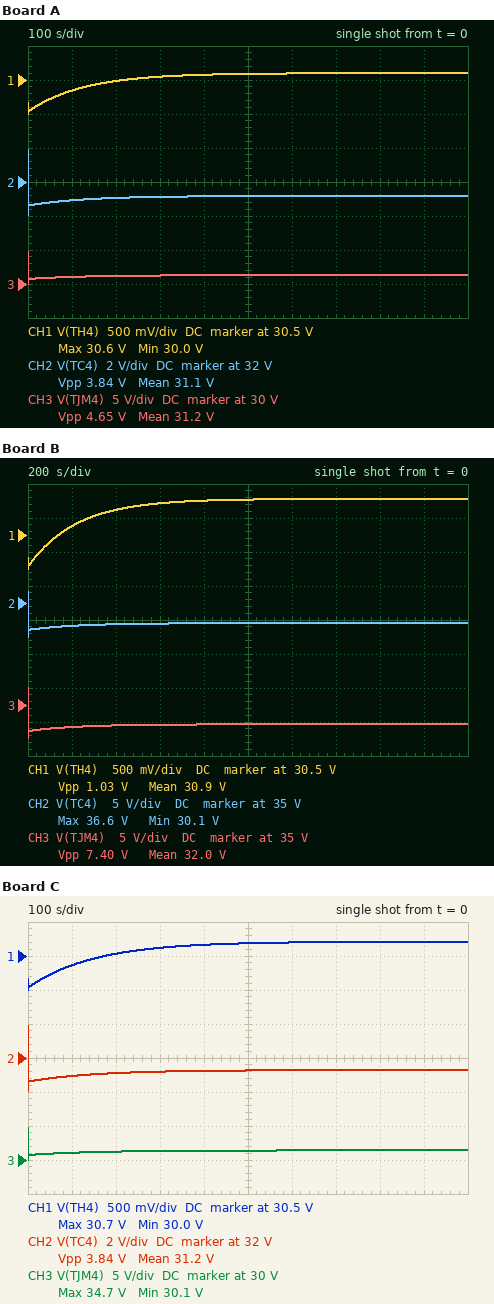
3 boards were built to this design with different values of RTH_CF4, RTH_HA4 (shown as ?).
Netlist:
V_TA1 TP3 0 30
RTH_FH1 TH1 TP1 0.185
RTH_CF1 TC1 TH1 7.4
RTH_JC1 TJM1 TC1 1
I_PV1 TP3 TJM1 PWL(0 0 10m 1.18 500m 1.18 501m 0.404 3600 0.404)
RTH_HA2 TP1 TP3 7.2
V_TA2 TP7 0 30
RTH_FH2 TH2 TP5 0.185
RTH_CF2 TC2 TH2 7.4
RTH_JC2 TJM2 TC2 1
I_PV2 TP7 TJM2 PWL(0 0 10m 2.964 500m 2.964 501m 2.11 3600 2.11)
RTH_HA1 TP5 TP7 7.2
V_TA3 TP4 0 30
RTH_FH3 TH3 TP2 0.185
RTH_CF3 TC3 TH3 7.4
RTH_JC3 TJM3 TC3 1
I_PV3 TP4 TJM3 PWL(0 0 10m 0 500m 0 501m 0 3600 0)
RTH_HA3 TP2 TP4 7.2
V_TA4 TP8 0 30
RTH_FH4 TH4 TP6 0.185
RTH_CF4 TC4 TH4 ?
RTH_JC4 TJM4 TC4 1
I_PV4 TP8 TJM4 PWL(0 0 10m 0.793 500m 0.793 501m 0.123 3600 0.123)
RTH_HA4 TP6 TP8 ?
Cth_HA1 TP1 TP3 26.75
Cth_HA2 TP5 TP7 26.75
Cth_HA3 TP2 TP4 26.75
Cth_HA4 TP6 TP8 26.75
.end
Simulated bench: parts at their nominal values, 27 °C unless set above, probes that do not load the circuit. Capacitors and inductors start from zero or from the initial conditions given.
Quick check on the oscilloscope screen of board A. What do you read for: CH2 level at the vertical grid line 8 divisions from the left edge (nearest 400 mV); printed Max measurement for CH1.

31.2 V
30.6 V
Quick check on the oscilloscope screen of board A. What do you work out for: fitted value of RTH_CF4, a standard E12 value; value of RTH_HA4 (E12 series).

4.7 Ω
4.7 Ω
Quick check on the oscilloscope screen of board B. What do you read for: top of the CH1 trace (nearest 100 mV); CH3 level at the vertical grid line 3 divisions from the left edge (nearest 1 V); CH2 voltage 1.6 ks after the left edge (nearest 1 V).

31.0 V
32 V
32 V
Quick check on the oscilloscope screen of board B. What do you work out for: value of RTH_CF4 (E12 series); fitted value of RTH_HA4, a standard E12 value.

8.2 Ω
8.2 Ω
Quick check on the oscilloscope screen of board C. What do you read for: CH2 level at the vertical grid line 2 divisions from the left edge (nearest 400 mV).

31.2 V
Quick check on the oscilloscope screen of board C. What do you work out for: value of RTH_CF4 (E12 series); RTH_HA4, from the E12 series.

4.7 Ω
5.6 Ω
